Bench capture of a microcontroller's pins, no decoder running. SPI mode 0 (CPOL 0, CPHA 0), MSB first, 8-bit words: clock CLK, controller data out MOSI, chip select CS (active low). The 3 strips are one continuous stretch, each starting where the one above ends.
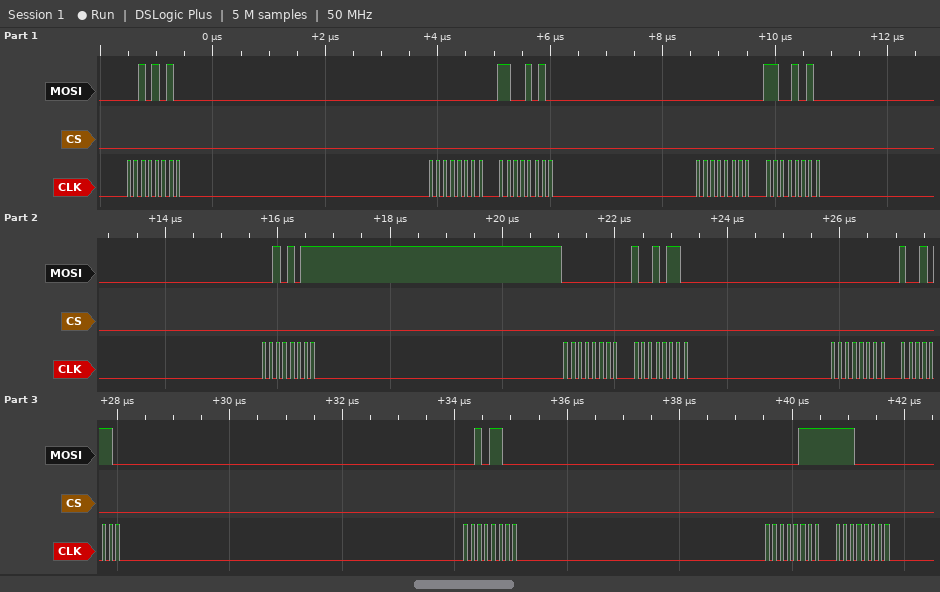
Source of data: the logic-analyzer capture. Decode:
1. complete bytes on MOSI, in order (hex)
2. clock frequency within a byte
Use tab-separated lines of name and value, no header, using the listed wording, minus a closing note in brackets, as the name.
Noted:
complete bytes on MOSI, in order	2A 00 CA 00 CA 2B 00 96 00 96 2C 07 E0
clock frequency within a byte	8 MHz
